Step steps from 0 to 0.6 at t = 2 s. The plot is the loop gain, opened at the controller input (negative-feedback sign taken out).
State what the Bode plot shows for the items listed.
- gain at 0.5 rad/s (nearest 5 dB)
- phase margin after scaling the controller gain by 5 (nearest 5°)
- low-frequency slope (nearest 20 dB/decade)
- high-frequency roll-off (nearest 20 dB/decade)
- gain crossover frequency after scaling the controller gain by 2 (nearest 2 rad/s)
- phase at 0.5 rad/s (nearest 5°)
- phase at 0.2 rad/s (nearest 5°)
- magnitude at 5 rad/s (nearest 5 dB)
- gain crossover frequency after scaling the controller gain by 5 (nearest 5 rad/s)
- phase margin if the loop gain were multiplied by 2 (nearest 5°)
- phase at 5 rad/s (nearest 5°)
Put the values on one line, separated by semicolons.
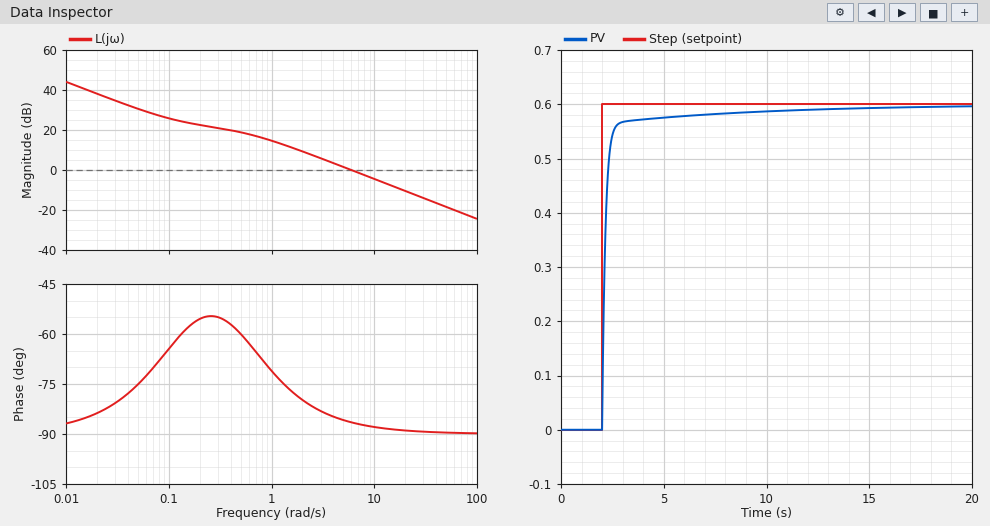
20 dB; 90°; -20 dB/decade; -20 dB/decade; 12 rad/s; -60°; -55°; 0 dB; 30 rad/s; 90°; -85°
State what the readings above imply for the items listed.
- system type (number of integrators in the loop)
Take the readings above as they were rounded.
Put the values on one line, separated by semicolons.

1
